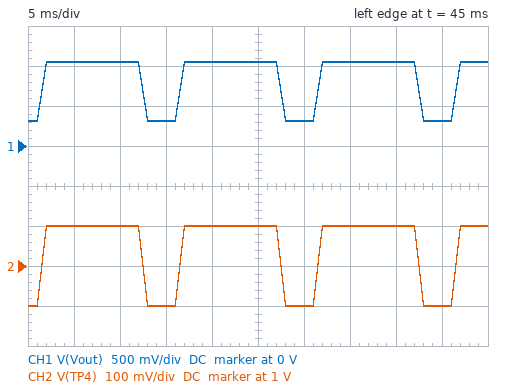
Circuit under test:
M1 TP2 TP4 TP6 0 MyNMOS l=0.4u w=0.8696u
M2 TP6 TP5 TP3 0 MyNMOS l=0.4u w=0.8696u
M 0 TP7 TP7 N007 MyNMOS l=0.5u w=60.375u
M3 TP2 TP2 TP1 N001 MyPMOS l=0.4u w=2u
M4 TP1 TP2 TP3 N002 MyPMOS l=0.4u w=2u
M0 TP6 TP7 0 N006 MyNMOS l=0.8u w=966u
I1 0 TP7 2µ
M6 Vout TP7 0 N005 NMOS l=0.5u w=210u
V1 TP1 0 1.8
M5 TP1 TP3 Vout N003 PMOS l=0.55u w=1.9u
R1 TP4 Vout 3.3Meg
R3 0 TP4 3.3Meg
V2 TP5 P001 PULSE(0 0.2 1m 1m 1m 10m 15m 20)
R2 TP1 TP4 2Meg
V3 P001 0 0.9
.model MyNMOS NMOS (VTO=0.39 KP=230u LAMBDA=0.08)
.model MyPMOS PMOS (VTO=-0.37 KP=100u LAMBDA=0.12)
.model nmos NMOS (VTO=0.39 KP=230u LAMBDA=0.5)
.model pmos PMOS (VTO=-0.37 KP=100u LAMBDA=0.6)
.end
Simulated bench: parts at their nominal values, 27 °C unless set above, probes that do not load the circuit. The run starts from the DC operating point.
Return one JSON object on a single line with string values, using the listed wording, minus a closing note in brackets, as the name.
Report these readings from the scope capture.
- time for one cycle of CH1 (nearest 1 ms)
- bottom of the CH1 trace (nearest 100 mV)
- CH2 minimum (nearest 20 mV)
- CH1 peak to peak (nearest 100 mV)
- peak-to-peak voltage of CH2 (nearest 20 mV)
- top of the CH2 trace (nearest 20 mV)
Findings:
{"time for one cycle of CH1": "15 ms", "bottom of the CH1 trace": "300 mV", "CH2 minimum": "900 mV", "CH1 peak to peak": "700 mV", "peak-to-peak voltage of CH2": "200 mV", "top of the CH2 trace": "1.10 V"}
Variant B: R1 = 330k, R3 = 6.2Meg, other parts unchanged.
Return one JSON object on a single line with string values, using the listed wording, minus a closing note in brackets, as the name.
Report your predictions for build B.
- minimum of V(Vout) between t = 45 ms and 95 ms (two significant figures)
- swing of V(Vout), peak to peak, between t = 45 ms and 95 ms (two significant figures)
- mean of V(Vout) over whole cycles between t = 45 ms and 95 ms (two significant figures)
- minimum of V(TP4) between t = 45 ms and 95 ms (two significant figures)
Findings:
{"minimum of V(Vout) between t = 45 ms and 95 ms": "800 mV", "swing of V(Vout), peak to peak, between t = 45 ms and 95 ms": "240 mV", "mean of V(Vout) over whole cycles between t = 45 ms and 95 ms": "980 mV", "minimum of V(TP4) between t = 45 ms and 95 ms": "900 mV"}
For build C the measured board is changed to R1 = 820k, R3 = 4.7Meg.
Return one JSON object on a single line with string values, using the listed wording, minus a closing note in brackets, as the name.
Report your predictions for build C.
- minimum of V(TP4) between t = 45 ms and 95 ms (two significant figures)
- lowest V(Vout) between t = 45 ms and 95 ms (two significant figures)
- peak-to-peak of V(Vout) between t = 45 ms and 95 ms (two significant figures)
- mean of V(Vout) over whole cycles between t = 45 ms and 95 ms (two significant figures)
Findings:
{"minimum of V(TP4) between t = 45 ms and 95 ms": "900 mV", "lowest V(Vout) between t = 45 ms and 95 ms": "690 mV", "peak-to-peak of V(Vout) between t = 45 ms and 95 ms": "320 mV", "mean of V(Vout) over whole cycles between t = 45 ms and 95 ms": "920 mV"}
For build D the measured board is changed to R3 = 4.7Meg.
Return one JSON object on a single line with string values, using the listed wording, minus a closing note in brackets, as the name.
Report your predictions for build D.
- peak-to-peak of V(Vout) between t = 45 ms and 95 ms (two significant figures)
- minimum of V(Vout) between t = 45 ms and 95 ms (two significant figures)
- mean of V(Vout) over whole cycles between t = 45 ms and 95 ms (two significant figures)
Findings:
{"peak-to-peak of V(Vout) between t = 45 ms and 95 ms": "670 mV", "minimum of V(Vout) between t = 45 ms and 95 ms": "50 mV", "mean of V(Vout) over whole cycles between t = 45 ms and 95 ms": "540 mV"}
